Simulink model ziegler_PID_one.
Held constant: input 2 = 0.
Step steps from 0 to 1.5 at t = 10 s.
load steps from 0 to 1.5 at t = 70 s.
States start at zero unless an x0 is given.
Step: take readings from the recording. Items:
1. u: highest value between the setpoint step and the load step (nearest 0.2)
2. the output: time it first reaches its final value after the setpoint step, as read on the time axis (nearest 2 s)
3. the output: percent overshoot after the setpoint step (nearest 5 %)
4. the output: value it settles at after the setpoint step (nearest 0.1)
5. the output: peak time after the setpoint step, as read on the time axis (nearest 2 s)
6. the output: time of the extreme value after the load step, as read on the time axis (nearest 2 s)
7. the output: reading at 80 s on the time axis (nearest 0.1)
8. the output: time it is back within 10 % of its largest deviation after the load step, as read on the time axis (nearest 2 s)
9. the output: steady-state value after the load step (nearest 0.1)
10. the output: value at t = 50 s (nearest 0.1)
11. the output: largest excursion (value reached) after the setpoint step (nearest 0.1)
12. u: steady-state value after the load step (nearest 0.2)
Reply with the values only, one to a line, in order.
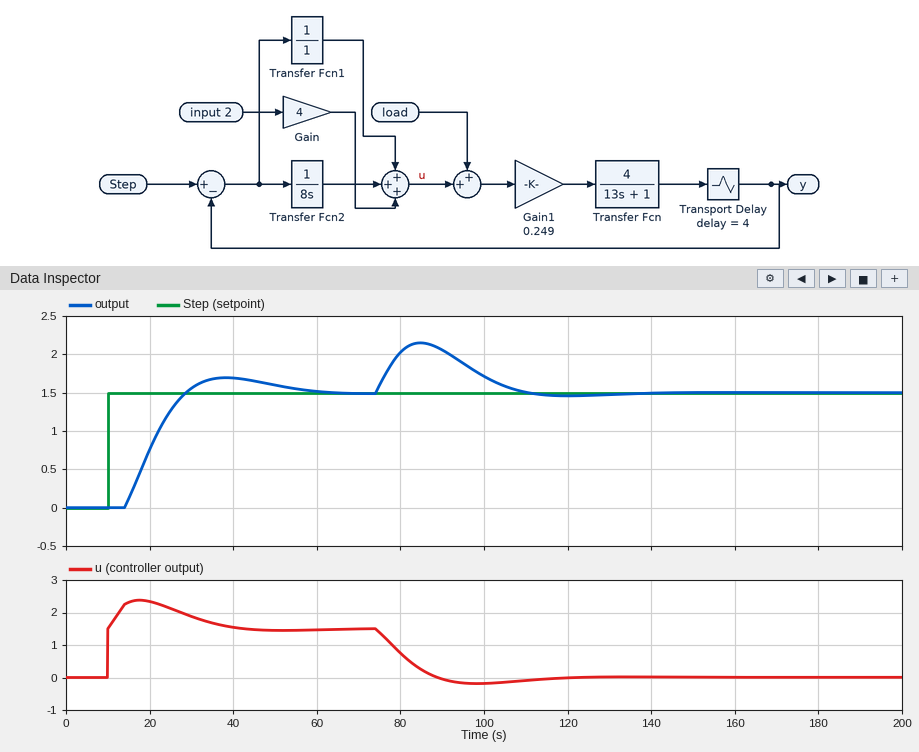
2.4
28 s
15 %
1.5
38 s
84 s
2.0
106 s
1.5
1.6
1.7
0.0
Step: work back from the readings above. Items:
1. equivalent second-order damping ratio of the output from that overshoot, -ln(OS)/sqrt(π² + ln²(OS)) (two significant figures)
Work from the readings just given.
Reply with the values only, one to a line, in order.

0.52
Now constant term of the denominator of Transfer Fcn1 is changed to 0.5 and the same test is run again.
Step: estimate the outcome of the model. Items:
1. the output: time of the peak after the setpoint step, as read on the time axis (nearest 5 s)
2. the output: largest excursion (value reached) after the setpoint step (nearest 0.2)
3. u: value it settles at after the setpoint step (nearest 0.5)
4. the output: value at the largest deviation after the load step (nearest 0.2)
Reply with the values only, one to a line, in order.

25 s
1.6
1.5
2.0
